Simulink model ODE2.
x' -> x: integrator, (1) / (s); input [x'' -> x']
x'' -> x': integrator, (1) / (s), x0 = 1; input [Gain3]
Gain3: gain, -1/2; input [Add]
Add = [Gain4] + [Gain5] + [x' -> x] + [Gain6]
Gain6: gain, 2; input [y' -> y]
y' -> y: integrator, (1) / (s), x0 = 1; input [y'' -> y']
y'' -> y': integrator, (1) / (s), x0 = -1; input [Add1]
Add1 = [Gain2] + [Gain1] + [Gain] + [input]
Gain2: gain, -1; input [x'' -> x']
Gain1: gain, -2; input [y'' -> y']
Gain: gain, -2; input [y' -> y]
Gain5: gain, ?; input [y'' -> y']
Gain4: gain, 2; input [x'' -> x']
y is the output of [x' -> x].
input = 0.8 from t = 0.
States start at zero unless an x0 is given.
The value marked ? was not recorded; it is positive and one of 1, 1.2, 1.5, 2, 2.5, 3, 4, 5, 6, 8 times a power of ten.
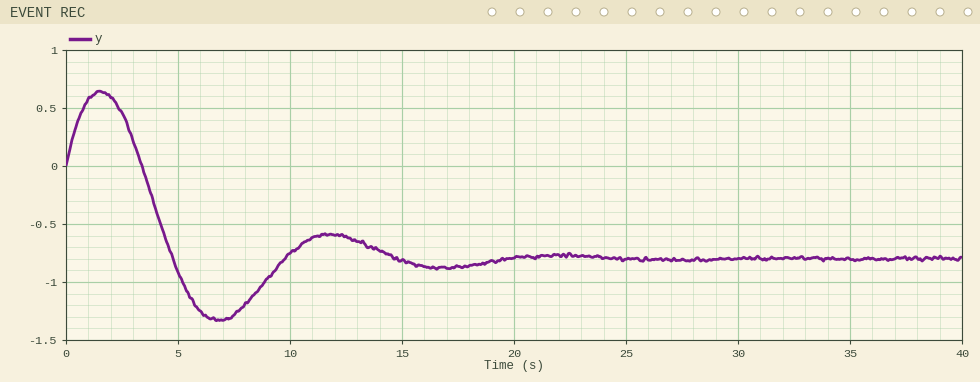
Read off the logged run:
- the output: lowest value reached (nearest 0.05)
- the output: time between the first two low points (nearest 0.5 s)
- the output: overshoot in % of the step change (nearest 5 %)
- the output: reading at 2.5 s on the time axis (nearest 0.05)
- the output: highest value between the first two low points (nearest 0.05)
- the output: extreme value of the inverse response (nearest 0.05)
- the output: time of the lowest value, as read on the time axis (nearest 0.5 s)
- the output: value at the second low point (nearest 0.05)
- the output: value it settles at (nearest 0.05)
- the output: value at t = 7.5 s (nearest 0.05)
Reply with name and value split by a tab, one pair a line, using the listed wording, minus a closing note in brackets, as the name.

the output: lowest value reached	-1.35
the output: time between the first two low points	10.0 s
the output: overshoot in % of the step change	65 %
the output: reading at 2.5 s on the time axis	0.45
the output: highest value between the first two low points	-0.60
the output: extreme value of the inverse response	0.65
the output: time of the lowest value, as read on the time axis	7.0 s
the output: value at the second low point	-0.90
the output: value it settles at	-0.80
the output: value at t = 7.5 s	-1.30
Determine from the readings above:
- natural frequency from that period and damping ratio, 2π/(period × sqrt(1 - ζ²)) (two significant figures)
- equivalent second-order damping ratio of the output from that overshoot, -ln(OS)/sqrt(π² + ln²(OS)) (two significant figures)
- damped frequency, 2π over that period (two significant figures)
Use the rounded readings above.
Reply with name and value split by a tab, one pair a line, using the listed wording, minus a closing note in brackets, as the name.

natural frequency from that period and damping ratio, 2π/(period × sqrt(1 - ζ²))	0.63 rad/s
equivalent second-order damping ratio of the output from that overshoot, -ln(OS)/sqrt(π² + ln²(OS))	0.14
damped frequency, 2π over that period	0.63 rad/s
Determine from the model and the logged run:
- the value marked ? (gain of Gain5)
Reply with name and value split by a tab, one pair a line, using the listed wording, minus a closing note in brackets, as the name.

the value marked ?	1.5
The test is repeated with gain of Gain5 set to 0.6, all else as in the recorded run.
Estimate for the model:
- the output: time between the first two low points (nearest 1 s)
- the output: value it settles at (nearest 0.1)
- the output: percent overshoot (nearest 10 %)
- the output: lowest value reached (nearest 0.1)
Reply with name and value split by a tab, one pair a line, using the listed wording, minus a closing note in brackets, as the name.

the output: time between the first two low points	11 s
the output: value it settles at	-0.8
the output: percent overshoot	50 %
the output: lowest value reached	-1.2
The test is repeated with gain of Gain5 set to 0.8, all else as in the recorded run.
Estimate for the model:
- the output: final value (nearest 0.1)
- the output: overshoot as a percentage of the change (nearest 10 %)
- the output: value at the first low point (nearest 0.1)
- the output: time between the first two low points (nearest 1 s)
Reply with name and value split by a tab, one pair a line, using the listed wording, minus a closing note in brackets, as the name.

the output: final value	-0.8
the output: overshoot as a percentage of the change	50 %
the output: value at the first low point	-1.2
the output: time between the first two low points	11 s
